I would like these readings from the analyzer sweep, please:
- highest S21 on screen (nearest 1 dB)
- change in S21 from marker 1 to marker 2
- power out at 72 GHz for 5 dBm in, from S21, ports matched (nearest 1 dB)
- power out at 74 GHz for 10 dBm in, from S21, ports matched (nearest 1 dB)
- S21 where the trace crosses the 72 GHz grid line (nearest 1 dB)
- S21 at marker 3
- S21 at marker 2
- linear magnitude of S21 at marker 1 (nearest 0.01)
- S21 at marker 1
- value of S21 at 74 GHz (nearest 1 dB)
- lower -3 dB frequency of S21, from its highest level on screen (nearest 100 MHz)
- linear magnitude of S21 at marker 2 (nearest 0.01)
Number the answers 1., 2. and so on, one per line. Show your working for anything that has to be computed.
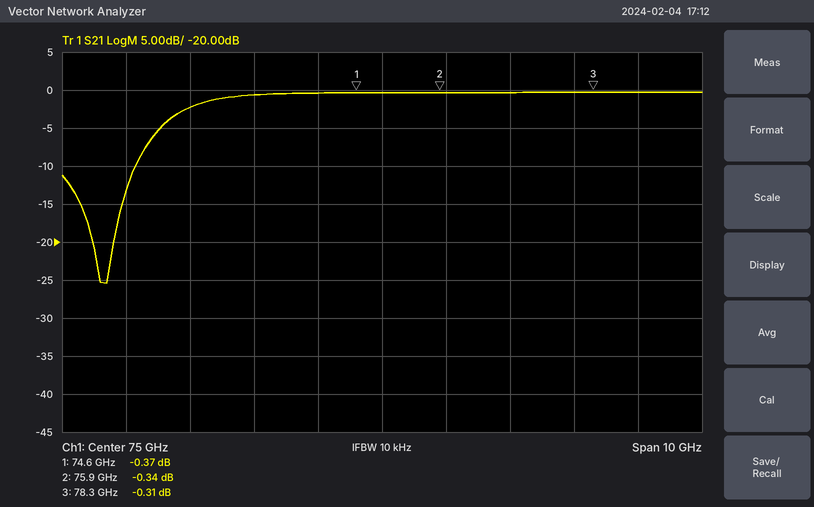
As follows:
1. 0 dB
2. -0.34 − (-0.37) = 0.03 dB
3. 5 dBm + (-2 dB) = 3 dBm
4. 10 dBm + (0 dB) = 10 dBm
5. -2 dB
6. -0.31 dB
7. -0.34 dB
8. 10^(-0.37/20) ≈ 0.96
9. -0.37 dB
10. 0 dB
11. 71.8 GHz
12. 10^(-0.34/20) ≈ 0.96
